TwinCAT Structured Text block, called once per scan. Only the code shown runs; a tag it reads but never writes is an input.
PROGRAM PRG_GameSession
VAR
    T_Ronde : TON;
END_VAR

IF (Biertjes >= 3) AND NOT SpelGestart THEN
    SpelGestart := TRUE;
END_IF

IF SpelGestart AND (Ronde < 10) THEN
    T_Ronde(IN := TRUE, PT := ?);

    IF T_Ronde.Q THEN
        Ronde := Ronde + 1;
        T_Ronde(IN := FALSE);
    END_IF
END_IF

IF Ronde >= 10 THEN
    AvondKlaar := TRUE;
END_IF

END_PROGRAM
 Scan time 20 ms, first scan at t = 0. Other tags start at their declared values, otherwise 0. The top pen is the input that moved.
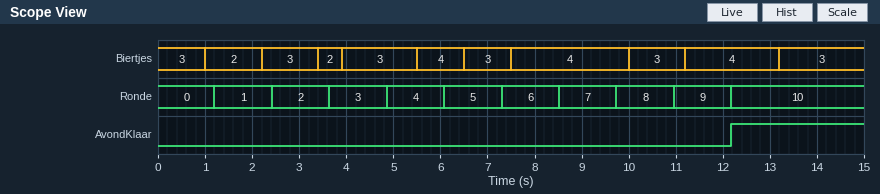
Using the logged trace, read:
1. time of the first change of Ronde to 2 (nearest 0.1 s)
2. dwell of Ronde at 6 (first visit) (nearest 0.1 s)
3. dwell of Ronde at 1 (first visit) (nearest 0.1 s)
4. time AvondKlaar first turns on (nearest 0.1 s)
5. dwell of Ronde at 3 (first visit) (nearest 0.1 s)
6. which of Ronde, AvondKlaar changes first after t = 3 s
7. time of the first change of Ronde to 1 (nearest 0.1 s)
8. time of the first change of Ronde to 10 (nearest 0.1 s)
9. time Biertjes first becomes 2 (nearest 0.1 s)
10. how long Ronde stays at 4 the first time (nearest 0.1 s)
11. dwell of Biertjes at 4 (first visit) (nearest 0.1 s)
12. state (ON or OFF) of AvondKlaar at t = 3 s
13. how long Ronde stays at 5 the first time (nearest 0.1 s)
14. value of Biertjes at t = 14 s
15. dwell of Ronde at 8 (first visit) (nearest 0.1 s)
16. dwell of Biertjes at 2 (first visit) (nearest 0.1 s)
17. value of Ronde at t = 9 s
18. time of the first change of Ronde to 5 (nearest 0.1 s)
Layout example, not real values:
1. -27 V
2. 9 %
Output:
1. 2.4 s
2. 1.2 s
3. 1.2 s
4. 12.2 s
5. 1.2 s
6. Ronde
7. 1.2 s
8. 12.2 s
9. 1.0 s
10. 1.2 s
11. 1.0 s
12. OFF
13. 1.2 s
14. 3
15. 1.2 s
16. 1.2 s
17. 7
18. 6.1 s
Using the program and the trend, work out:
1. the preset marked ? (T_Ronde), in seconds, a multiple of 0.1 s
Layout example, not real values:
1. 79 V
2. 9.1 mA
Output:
1. 1.2 s
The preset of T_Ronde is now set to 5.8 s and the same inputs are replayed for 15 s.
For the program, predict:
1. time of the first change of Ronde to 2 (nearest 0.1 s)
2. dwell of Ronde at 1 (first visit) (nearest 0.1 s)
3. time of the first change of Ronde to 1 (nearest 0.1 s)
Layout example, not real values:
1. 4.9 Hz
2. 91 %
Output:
1. 11.6 s
2. 5.8 s
3. 5.8 s
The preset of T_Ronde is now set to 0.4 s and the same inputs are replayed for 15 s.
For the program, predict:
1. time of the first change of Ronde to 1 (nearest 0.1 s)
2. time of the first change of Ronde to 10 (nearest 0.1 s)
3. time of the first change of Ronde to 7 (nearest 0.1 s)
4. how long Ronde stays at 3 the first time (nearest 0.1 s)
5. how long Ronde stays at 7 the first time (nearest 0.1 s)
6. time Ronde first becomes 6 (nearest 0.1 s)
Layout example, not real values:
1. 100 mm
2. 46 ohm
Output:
1. 0.4 s
2. 4.2 s
3. 2.9 s
4. 0.4 s
5. 0.4 s
6. 2.5 s
